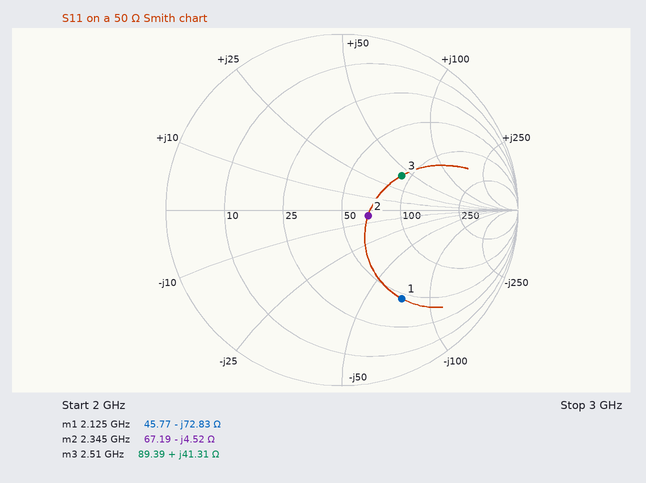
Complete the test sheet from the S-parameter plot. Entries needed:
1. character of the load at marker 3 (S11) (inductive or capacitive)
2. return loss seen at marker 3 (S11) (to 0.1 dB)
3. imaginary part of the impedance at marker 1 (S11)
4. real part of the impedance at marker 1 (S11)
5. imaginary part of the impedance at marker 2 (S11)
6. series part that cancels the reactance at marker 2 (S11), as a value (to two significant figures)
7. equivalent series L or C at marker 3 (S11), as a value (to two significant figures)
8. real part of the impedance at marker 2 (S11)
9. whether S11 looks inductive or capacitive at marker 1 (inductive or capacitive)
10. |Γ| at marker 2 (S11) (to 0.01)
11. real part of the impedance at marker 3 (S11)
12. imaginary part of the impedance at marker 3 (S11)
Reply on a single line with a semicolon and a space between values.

inductive; 8.1 dB; -72.83 Ω; 45.77 Ω; -4.52 Ω; 310 pH; 2.6 nH; 67.19 Ω; capacitive; 0.15; 89.39 Ω; +41.31 Ω
